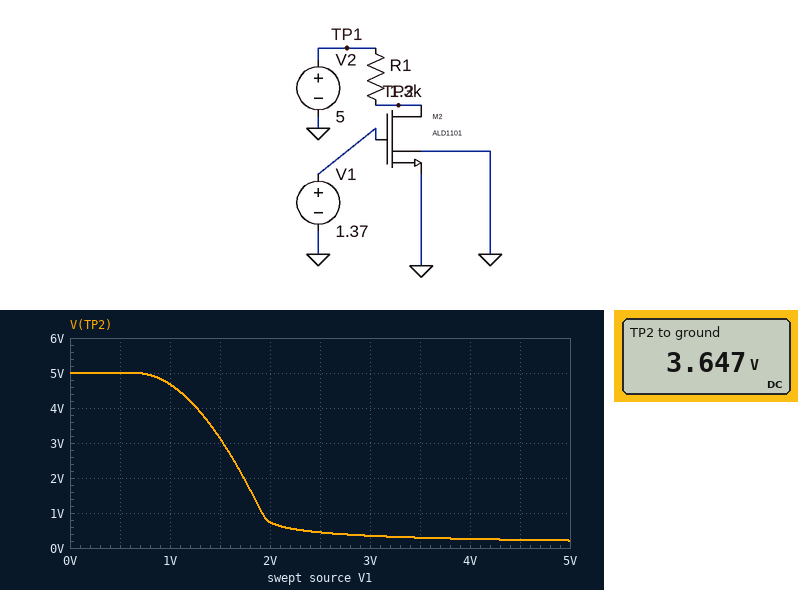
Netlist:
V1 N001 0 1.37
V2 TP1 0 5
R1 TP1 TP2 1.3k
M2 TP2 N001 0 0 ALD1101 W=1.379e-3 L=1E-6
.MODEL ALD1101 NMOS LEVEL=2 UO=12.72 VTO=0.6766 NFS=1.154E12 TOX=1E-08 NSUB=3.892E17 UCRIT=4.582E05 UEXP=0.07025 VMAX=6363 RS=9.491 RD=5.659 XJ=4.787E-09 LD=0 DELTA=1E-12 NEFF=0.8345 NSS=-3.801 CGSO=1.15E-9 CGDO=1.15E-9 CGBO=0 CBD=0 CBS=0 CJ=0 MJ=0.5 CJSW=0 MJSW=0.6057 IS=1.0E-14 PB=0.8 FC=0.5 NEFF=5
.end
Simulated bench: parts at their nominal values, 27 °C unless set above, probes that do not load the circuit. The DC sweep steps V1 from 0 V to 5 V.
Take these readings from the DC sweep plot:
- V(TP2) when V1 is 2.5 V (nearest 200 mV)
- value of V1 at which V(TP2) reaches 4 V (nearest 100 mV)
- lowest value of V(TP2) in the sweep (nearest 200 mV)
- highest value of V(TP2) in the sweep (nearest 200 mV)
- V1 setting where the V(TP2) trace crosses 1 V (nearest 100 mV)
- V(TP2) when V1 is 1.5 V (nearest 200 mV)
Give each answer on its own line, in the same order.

400 mV
1.3 V
200 mV
5.0 V
1.9 V
3.2 V
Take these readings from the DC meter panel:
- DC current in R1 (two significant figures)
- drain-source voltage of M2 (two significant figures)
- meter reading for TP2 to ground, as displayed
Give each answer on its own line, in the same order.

1.0 mA
3.6 V
3.647 V
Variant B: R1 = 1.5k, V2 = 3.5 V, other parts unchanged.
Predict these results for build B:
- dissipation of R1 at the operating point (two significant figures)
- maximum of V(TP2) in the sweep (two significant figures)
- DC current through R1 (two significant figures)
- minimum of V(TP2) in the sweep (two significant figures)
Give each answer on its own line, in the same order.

1.6 mW
3.5 V
1.0 mA
130 mV
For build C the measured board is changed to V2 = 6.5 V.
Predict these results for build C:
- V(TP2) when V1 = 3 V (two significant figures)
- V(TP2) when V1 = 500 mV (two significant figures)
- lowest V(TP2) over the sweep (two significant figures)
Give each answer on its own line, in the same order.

470 mV
6.5 V
280 mV
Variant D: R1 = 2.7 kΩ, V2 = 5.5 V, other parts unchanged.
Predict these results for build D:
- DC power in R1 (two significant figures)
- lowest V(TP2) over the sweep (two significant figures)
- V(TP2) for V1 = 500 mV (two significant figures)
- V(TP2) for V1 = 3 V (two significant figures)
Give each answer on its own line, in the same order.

2.9 mW
110 mV
5.5 V
180 mV
